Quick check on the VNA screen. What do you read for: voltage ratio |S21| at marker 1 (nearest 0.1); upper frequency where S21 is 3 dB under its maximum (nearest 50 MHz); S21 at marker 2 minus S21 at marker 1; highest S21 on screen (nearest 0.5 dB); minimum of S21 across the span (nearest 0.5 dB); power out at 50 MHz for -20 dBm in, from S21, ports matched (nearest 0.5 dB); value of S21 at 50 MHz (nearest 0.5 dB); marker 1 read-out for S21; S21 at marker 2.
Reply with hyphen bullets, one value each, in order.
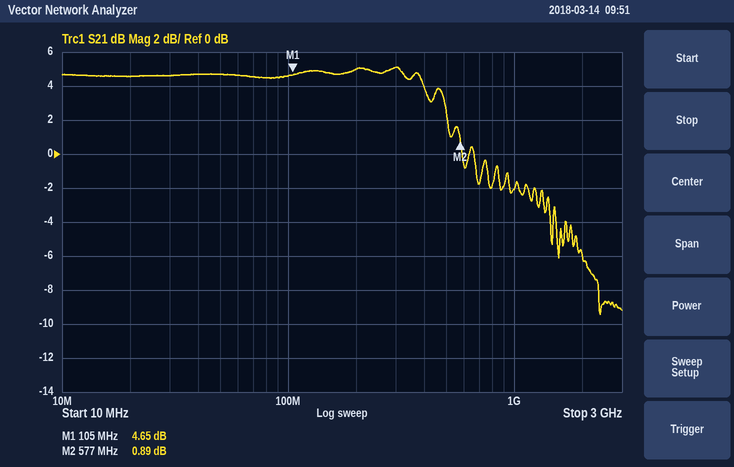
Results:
- 1.7
- 500 MHz
- -3.76 dB
- 5.0 dB
- -9.5 dB
- -15.5 dBm
- 4.5 dB
- 4.65 dB
- 0.89 dB
